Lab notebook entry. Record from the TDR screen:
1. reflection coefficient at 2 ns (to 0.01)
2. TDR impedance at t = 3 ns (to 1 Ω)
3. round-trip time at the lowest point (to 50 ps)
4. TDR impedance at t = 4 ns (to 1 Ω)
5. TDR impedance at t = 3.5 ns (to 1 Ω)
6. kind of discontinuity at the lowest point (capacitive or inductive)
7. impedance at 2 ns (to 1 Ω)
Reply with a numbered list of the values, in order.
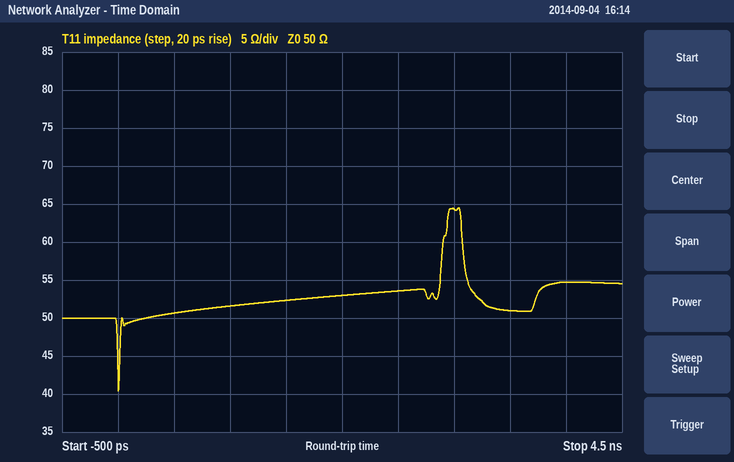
1. +0.03
2. 64 Ω
3. 0 ps
4. 55 Ω
5. 51 Ω
6. capacitive
7. 53 Ω
